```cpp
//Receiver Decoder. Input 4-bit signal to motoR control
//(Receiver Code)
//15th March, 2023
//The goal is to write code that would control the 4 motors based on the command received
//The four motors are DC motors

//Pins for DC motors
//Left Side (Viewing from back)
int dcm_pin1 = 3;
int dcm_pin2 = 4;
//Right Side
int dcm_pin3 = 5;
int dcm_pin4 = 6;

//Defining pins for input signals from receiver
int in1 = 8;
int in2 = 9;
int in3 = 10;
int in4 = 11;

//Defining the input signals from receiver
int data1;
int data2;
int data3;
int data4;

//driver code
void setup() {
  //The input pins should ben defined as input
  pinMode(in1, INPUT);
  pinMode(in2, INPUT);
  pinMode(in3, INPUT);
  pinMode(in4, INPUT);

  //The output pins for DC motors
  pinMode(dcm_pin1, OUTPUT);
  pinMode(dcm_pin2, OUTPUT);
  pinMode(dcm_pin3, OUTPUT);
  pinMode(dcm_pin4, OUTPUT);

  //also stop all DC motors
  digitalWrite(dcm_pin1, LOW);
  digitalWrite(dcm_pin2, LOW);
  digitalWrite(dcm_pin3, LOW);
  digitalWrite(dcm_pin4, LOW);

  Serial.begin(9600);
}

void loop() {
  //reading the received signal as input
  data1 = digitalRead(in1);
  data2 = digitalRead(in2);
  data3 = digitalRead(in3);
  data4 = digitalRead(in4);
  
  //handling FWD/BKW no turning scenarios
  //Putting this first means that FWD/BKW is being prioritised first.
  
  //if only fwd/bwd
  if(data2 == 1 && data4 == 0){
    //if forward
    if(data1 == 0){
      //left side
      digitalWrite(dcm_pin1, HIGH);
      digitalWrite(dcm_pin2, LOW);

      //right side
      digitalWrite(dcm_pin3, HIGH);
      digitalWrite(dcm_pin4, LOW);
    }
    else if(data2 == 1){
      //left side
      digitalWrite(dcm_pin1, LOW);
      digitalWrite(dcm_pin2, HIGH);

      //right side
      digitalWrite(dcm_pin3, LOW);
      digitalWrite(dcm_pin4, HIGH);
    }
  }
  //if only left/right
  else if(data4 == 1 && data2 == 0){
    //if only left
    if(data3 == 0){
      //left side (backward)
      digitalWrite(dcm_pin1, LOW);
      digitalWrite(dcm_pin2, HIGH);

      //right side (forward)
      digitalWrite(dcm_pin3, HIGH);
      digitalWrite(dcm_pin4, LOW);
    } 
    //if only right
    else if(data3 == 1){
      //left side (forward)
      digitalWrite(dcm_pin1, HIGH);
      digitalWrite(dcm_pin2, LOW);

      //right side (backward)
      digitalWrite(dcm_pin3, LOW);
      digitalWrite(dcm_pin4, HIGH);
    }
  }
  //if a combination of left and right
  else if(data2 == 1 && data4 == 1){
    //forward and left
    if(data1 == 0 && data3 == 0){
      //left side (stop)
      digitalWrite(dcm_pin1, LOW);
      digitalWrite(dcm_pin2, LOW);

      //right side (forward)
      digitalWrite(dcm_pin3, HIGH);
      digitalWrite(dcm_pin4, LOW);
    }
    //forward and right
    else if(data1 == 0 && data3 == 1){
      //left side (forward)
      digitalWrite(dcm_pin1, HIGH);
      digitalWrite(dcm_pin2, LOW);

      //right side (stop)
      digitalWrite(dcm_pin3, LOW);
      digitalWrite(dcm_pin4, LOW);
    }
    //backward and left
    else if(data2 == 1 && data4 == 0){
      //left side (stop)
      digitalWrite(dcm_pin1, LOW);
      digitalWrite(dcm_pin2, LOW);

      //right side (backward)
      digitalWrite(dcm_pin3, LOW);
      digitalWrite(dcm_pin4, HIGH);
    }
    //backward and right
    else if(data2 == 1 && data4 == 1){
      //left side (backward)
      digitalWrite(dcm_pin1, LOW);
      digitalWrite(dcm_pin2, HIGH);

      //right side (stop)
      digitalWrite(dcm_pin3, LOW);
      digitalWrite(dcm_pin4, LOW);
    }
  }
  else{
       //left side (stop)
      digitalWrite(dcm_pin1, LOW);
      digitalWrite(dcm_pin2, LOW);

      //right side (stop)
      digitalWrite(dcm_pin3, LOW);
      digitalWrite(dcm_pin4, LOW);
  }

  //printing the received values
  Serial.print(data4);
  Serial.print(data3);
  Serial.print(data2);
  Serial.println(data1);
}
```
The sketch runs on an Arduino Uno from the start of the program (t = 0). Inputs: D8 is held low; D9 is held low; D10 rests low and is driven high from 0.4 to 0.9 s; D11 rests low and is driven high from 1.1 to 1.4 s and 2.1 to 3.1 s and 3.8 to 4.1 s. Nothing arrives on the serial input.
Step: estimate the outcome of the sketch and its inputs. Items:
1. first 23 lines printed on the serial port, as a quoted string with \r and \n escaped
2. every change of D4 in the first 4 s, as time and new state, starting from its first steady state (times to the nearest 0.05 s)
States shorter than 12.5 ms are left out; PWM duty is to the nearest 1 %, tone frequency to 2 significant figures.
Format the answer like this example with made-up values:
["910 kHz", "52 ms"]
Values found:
["\"0000\\r\\n0000\\r\\n0000\\r\\n0000\\r\\n0000\\r\\n0000\\r\\n0000\\r\\n0000\\r\\n0000\\r\\n0000\\r\\n0000\\r\\n0000\\r\\n0000\\r\\n0000\\r\\n0000\\r\\n0000\\r\\n0000\\r\\n0000\\r\\n0000\\r\\n0000\\r\\n0000\\r\\n0000\\r\\n0000\\r\\n\"", "0 s low; 1.1 s high; 1.4 s low; 2.1 s high; 3.1 s low; 3.8 s high"]
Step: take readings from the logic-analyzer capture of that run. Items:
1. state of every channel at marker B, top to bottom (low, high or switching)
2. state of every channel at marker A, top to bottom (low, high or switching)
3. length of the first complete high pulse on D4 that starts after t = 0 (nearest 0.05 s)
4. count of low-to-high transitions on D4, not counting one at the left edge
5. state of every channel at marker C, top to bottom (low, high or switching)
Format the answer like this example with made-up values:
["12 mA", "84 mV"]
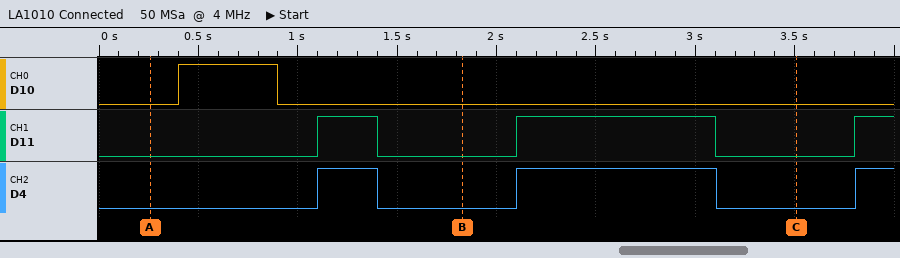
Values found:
["D10 low, D11 low, D4 low", "D10 low, D11 low, D4 low", "0.30 s", "3", "D10 low, D11 low, D4 low"]
